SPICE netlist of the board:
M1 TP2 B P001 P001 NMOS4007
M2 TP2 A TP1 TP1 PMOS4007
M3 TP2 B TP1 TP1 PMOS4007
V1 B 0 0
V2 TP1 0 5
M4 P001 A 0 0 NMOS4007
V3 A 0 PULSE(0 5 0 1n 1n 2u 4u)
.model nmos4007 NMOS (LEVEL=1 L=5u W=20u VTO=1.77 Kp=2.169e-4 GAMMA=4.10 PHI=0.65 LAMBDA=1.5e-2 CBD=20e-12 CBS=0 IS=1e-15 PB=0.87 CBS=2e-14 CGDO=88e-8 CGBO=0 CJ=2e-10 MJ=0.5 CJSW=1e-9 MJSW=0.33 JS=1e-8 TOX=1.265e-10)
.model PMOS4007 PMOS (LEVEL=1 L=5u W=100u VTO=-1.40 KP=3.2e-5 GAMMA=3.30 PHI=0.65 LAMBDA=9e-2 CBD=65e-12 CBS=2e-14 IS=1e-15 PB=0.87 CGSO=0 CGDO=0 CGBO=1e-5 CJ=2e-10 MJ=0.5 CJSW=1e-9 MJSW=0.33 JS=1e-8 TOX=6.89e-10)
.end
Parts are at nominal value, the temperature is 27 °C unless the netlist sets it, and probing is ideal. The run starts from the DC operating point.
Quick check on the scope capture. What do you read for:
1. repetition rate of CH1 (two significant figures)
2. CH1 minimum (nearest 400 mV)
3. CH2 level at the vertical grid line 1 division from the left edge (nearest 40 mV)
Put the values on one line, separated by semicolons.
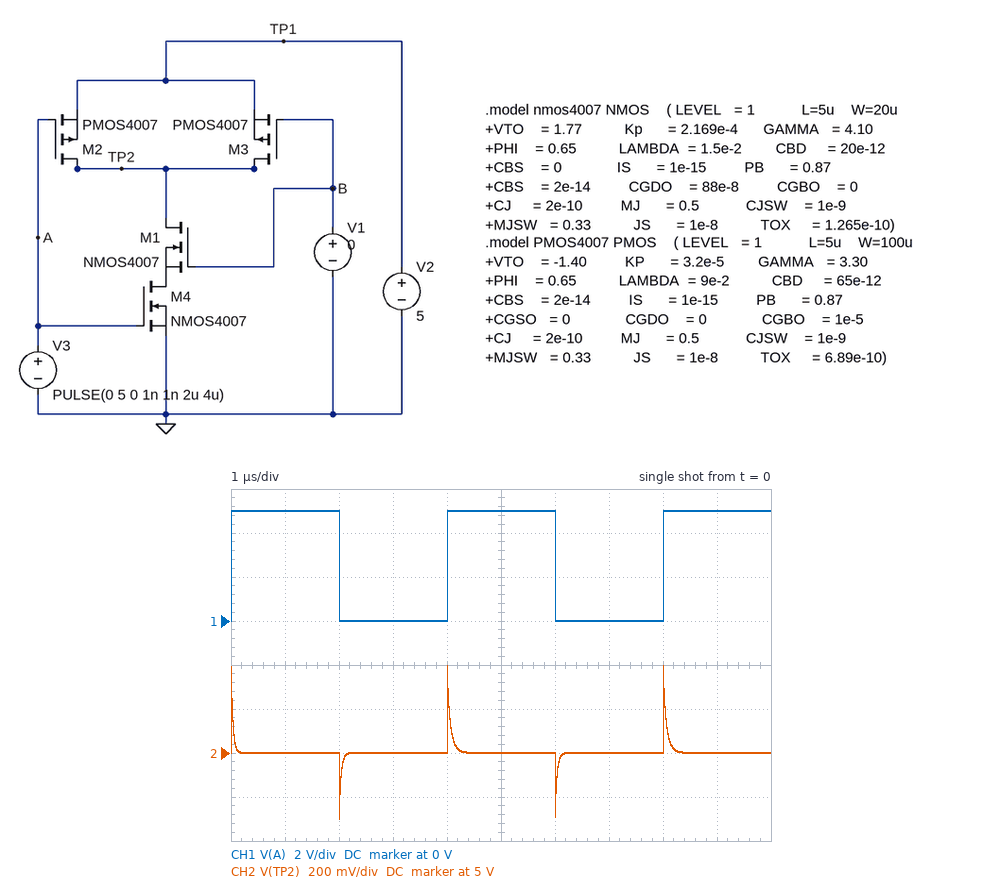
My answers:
250 kHz; 0 V; 5.00 V
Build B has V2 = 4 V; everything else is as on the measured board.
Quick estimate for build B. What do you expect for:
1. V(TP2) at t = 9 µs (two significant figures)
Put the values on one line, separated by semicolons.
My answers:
4.0 V
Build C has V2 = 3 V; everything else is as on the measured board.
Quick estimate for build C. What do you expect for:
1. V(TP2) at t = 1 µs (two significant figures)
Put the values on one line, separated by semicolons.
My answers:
3.0 V
